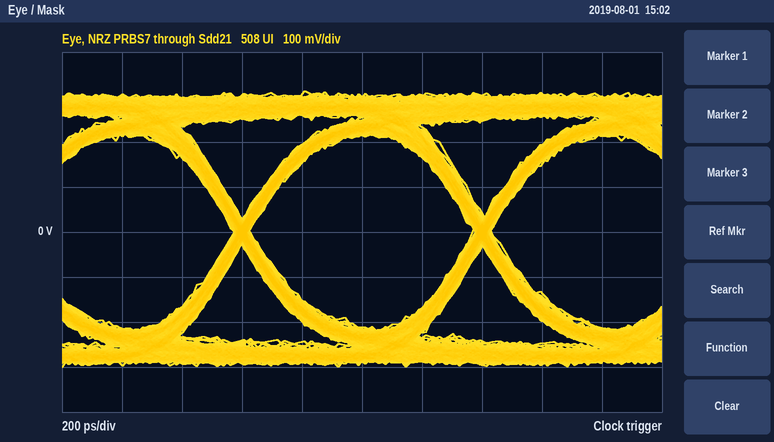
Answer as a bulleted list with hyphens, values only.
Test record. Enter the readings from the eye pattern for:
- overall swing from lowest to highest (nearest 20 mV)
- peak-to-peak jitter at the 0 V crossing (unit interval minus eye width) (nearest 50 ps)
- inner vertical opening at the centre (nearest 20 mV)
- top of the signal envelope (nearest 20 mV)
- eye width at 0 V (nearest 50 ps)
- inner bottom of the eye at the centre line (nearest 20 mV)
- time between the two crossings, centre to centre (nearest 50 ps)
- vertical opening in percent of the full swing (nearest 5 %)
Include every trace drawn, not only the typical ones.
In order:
- 620 mV
- 50 ps
- 420 mV
- 320 mV
- 750 ps
- -220 mV
- 800 ps
- 70 %
